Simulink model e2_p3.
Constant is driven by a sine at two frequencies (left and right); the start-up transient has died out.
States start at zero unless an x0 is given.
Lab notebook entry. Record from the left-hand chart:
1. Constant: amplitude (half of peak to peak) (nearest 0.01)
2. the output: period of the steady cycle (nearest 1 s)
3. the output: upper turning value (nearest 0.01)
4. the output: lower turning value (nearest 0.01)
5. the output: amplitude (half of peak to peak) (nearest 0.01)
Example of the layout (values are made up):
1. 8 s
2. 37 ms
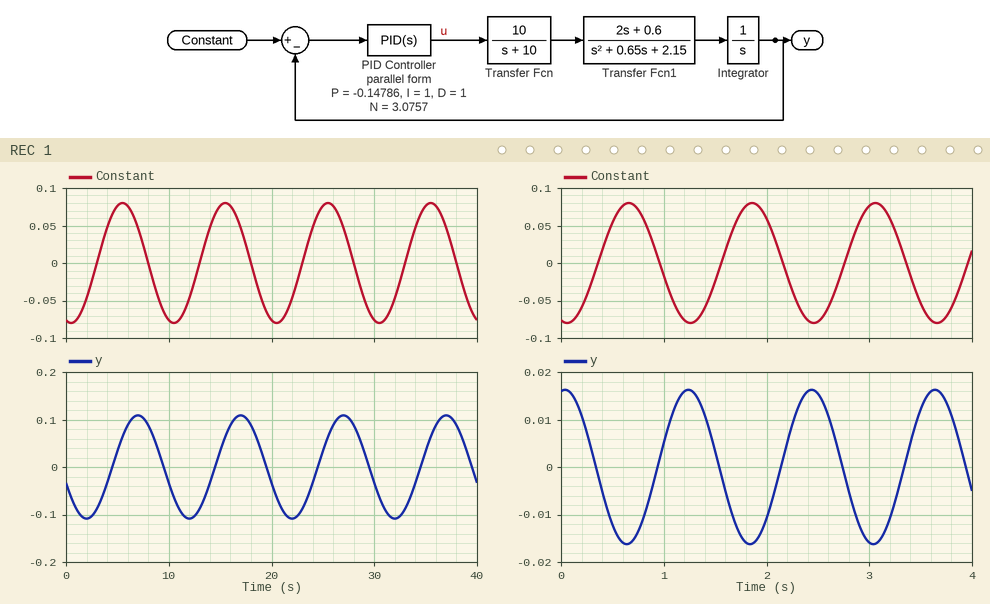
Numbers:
1. 0.08
2. 10 s
3. 0.11
4. -0.11
5. 0.11
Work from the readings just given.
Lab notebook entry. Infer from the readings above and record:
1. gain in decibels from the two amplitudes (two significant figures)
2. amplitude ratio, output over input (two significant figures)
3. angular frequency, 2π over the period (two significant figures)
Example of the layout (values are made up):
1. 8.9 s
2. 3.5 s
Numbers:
1. 2.8 dB
2. 1.4
3. 0.63 rad/s
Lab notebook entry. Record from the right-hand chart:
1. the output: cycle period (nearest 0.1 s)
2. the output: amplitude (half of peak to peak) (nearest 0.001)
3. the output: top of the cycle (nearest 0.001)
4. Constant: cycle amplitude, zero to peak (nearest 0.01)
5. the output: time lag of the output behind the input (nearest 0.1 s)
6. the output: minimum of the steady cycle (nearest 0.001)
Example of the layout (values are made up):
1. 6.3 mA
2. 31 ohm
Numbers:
1. 1.2 s
2. 0.016
3. 0.016
4. 0.08
5. 0.6 s
6. -0.016
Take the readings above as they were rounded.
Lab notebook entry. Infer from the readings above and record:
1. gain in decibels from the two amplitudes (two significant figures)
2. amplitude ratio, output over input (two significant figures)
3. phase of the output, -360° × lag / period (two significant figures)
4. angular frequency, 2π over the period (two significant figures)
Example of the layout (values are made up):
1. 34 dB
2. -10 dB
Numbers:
1. -14 dB
2. 0.20
3. -180°
4. 5.2 rad/s
